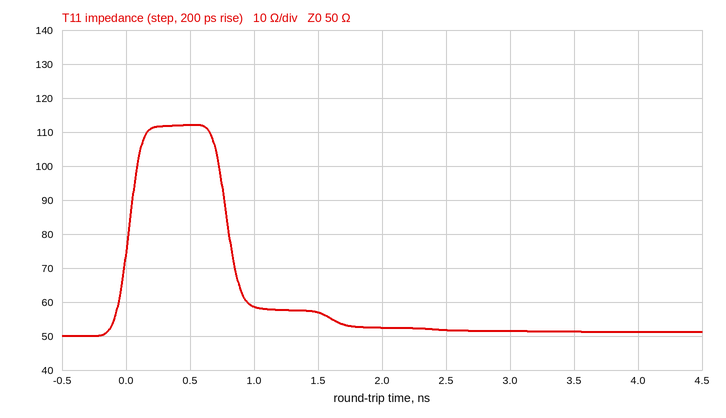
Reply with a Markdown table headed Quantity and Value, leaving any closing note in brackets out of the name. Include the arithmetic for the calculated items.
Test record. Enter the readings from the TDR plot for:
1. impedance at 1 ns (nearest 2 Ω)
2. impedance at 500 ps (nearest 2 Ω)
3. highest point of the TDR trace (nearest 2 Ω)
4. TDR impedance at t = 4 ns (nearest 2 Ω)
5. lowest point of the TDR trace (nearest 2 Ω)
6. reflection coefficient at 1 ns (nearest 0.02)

| Quantity | Value |
|---|---|
| impedance at 1 ns | 58 Ω |
| impedance at 500 ps | 112 Ω |
| highest point of the TDR trace | 112 Ω |
| TDR impedance at t = 4 ns | 52 Ω |
| lowest point of the TDR trace | 50 Ω |
| reflection coefficient at 1 ns | (58 − 50)/(58 + 50) ≈ +0.0741, so +0.08 to the nearest 0.02 |
